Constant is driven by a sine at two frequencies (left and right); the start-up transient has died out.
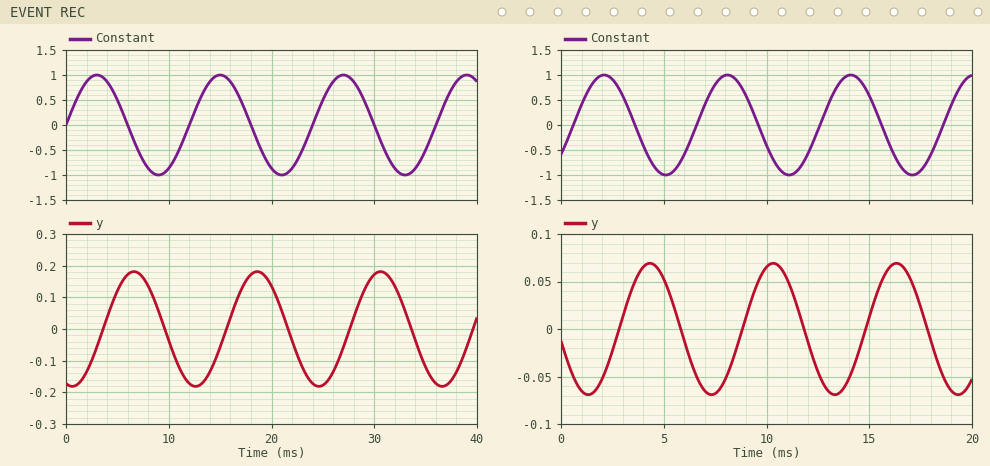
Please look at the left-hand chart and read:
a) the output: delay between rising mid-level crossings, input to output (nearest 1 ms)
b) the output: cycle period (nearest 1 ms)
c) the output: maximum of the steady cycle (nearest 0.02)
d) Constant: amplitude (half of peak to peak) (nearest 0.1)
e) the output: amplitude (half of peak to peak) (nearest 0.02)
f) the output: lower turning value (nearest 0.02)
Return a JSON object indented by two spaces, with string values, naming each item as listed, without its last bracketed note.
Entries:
{
  "the output: delay between rising mid-level crossings, input to output": "4 ms",
  "the output: cycle period": "12 ms",
  "the output: maximum of the steady cycle": "0.18",
  "Constant: amplitude (half of peak to peak)": "1.0",
  "the output: amplitude (half of peak to peak)": "0.18",
  "the output: lower turning value": "-0.18"
}
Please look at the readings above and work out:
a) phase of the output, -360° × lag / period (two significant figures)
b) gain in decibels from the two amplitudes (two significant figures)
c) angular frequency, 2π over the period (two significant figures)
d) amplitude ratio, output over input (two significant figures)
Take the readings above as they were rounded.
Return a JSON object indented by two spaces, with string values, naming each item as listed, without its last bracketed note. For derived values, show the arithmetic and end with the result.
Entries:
{
  "phase of the output, -360° × lag / period": "-360 × 4 / 12 = -120°",
  "gain in decibels from the two amplitudes": "20 log10(0.18 / 1) = -15 dB",
  "angular frequency, 2π over the period": "2π / 12 = 0.52 rad/ms",
  "amplitude ratio, output over input": "0.18 / 1 = 0.18"
}
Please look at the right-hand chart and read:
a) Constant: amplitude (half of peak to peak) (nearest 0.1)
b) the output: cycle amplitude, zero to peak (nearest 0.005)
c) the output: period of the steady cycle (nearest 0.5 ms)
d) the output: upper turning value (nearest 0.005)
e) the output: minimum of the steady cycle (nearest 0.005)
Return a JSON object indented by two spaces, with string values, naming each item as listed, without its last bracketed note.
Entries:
{
  "Constant: amplitude (half of peak to peak)": "1.0",
  "the output: cycle amplitude, zero to peak": "0.070",
  "the output: period of the steady cycle": "6.0 ms",
  "the output: upper turning value": "0.070",
  "the output: minimum of the steady cycle": "-0.070"
}
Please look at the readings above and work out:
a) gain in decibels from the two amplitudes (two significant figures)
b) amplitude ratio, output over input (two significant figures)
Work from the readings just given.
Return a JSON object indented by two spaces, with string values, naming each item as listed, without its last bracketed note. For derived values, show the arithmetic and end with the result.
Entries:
{
  "gain in decibels from the two amplitudes": "20 log10(0.07 / 1) = -23 dB",
  "amplitude ratio, output over input": "0.07 / 1 = 0.070"
}
